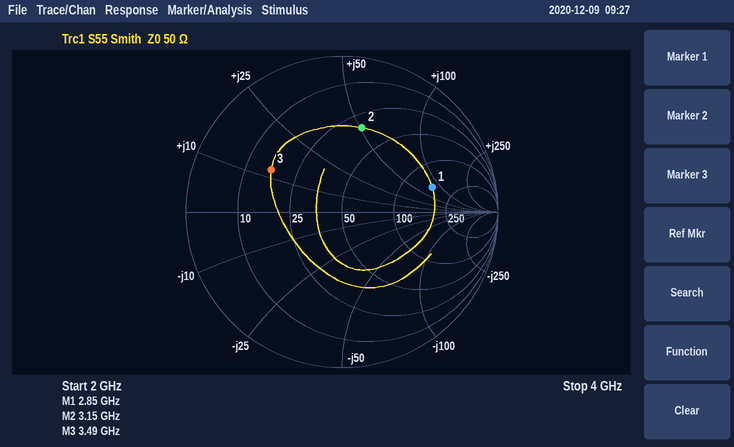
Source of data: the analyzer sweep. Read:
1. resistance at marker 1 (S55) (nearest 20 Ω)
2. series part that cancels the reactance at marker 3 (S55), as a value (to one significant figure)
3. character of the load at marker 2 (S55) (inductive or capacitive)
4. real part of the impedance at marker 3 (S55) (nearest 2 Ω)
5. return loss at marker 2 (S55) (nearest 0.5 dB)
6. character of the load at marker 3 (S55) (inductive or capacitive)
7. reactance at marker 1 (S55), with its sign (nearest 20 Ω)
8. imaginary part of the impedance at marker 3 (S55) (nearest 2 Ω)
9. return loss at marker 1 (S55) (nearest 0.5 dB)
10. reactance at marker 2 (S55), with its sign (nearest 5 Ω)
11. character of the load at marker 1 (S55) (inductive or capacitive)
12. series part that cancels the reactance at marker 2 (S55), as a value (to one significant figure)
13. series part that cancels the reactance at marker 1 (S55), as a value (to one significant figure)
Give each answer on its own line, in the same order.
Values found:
160 Ω
4 pF
inductive
16 Ω
5.0 dB
inductive
+80 Ω
+12 Ω
4.5 dB
+50 Ω
inductive
1.0 pF
700 fF
